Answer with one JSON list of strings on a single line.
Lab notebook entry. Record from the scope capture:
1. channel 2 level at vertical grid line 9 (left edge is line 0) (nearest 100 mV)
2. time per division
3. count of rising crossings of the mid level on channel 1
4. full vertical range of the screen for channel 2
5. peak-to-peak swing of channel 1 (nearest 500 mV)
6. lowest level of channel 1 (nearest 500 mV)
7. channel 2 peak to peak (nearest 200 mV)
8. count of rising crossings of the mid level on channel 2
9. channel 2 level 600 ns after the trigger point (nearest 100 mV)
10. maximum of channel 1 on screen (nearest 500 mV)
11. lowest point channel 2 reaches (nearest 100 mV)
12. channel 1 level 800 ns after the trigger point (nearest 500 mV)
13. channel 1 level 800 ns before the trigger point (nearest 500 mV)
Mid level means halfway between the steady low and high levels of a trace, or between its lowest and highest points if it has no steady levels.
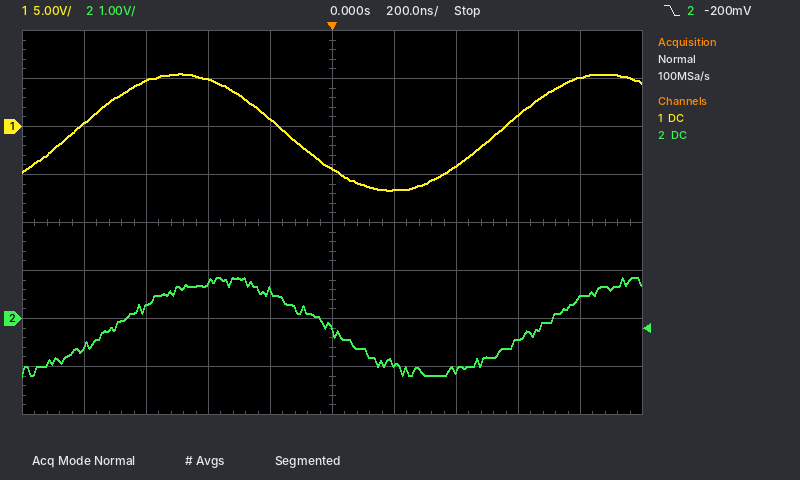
["400 mV", "200 ns", "2", "8 V", "12.0 V", "-6.5 V", "2.0 V", "2", "-400 mV", "5.5 V", "-1.2 V", "5.0 V", "500 mV"]
